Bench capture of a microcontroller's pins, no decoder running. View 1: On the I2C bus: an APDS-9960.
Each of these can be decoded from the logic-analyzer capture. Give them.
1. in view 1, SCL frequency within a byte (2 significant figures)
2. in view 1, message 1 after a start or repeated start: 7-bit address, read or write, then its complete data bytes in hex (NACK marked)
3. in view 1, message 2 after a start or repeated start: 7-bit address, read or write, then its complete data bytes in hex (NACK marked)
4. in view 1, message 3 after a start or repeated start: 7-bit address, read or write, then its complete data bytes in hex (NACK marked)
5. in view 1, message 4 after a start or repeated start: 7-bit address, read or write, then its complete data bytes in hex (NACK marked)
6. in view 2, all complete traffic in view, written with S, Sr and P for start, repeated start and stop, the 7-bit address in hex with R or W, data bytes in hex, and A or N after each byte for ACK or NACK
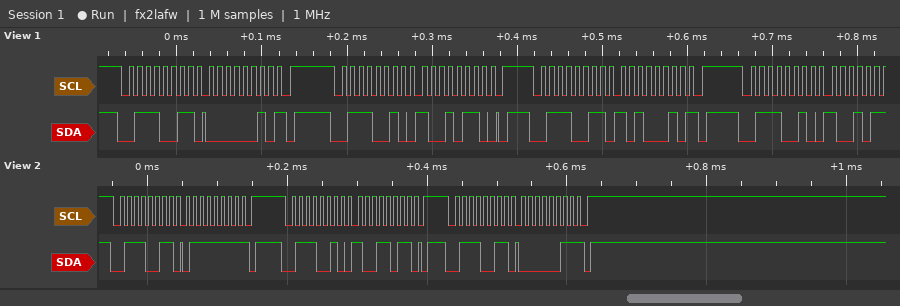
100 kHz
0x39 read: 02 NACK
0x39 write: 96
0x39 read: A2 NACK
0x39 write
S 39R A 7F N P S 39W A 9B A P S 39R A 03 N P
